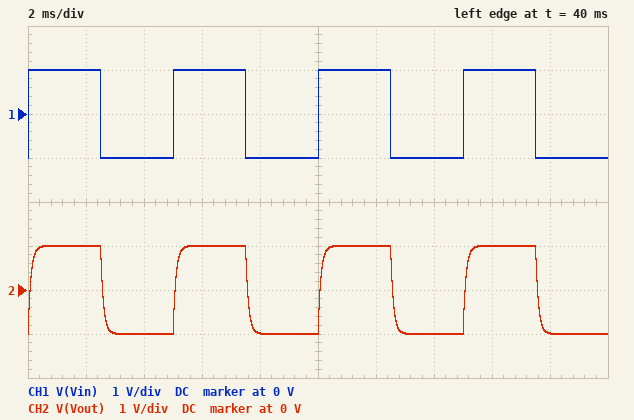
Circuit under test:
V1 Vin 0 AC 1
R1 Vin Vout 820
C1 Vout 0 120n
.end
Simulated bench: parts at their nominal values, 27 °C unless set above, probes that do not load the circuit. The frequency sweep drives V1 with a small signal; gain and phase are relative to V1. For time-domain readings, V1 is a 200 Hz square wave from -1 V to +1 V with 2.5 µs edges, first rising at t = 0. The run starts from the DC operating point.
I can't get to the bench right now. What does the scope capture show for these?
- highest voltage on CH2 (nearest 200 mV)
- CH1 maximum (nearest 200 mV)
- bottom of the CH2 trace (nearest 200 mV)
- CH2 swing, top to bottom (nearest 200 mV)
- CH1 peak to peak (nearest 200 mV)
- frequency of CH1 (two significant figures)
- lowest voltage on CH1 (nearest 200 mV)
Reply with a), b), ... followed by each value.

a) 1.0 V
b) 1.0 V
c) -1.0 V
d) 2.0 V
e) 2.0 V
f) 200 Hz
g) -1.0 V
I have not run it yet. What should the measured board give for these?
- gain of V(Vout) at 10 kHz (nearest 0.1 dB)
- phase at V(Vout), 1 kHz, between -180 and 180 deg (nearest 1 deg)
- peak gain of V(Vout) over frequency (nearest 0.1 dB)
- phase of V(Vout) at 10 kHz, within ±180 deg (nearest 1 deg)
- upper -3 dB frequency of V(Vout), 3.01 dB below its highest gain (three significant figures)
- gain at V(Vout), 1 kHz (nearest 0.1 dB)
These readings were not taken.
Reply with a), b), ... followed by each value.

a) -15.9 dB
b) -32 deg
c) 0 dB
d) -81 deg
e) 1.62 kHz
f) -1.4 dB
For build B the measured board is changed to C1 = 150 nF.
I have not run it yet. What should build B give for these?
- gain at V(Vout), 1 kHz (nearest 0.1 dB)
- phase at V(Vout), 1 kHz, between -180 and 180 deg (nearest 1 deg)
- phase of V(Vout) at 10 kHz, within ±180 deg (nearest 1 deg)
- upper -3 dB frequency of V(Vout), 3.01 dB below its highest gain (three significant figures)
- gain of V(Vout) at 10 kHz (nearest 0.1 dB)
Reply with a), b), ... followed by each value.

a) -2.0 dB
b) -38 deg
c) -83 deg
d) 1.29 kHz
e) -17.8 dB
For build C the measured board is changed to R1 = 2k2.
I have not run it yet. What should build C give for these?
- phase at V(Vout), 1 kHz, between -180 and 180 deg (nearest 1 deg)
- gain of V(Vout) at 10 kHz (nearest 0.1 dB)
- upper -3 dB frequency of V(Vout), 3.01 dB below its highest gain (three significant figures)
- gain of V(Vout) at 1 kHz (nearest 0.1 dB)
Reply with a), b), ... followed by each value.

a) -59 deg
b) -24.4 dB
c) 603 Hz
d) -5.7 dB
